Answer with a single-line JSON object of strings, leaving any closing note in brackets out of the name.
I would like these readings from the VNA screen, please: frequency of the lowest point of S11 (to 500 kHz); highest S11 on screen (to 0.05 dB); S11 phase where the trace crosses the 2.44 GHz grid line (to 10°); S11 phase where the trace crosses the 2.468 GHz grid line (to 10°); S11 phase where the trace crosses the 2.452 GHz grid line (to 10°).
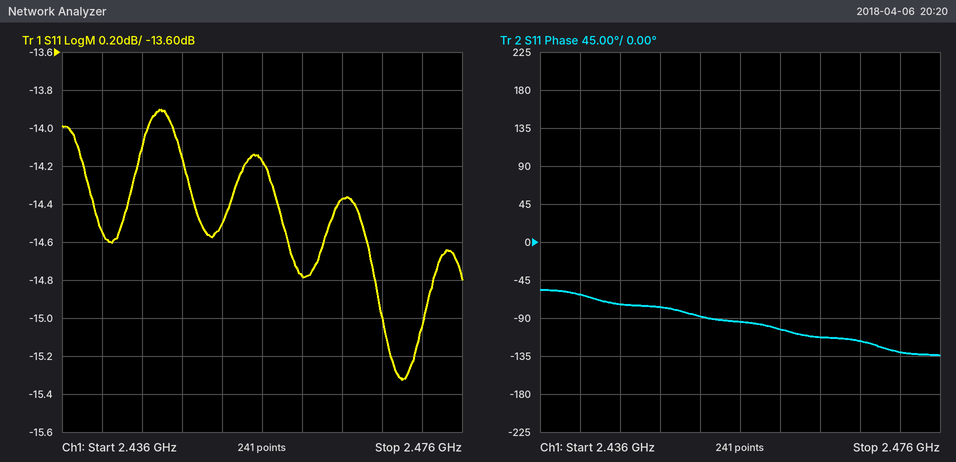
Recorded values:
{"frequency of the lowest point of S11": "2.4700 GHz", "highest S11 on screen": "-13.90 dB", "S11 phase where the trace crosses the 2.44 GHz grid line": "-60°", "S11 phase where the trace crosses the 2.468 GHz grid line": "-120°", "S11 phase where the trace crosses the 2.452 GHz grid line": "-90°"}
